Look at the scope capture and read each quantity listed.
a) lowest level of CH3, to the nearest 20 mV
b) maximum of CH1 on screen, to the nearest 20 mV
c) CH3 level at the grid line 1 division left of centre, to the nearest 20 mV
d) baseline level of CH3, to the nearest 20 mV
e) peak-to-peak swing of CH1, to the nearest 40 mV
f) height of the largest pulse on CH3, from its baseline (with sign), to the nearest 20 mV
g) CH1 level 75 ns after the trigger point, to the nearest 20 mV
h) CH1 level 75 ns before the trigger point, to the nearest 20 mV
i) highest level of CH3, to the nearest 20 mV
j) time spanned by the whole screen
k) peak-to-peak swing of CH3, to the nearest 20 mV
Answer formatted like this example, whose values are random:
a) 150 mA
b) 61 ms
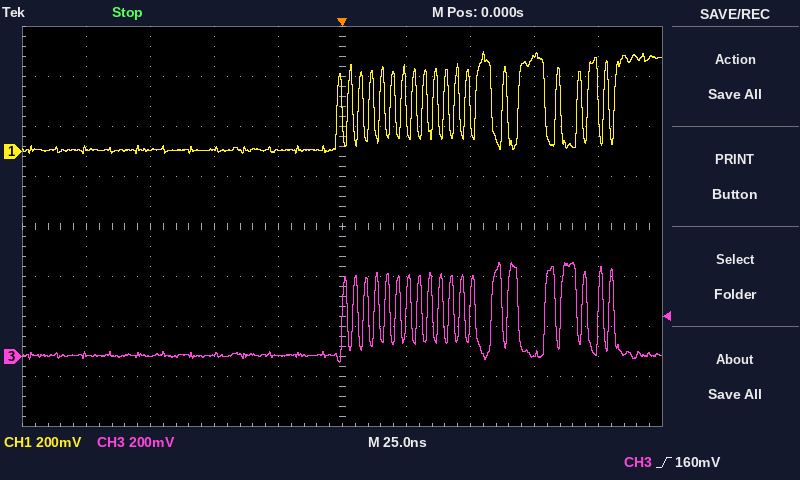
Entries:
a) -20 mV
b) 400 mV
c) 0 mV
d) 0 mV
e) 400 mV
f) +380 mV
g) 380 mV
h) 0 mV
i) 380 mV
j) 250 ns
k) 400 mV
